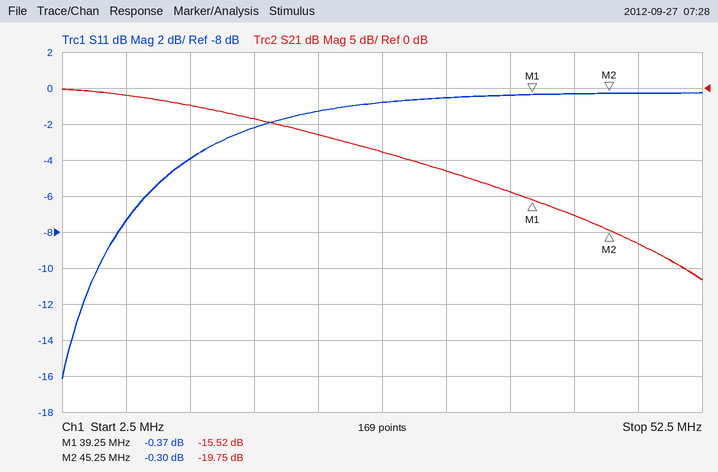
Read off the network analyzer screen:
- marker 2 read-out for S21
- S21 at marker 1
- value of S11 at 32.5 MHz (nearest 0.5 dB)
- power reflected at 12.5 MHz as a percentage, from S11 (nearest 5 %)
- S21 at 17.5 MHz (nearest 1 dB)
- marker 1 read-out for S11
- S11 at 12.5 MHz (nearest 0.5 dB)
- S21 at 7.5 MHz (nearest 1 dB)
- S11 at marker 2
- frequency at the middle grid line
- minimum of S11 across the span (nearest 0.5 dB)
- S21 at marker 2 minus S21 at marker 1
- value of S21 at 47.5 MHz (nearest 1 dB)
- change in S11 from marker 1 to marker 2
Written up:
-19.75 dB
-15.52 dB
-0.5 dB
40 %
-4 dB
-0.37 dB
-4.0 dB
-1 dB
-0.30 dB
27.5 MHz
-16.0 dB
-4.23 dB
-22 dB
0.07 dB
